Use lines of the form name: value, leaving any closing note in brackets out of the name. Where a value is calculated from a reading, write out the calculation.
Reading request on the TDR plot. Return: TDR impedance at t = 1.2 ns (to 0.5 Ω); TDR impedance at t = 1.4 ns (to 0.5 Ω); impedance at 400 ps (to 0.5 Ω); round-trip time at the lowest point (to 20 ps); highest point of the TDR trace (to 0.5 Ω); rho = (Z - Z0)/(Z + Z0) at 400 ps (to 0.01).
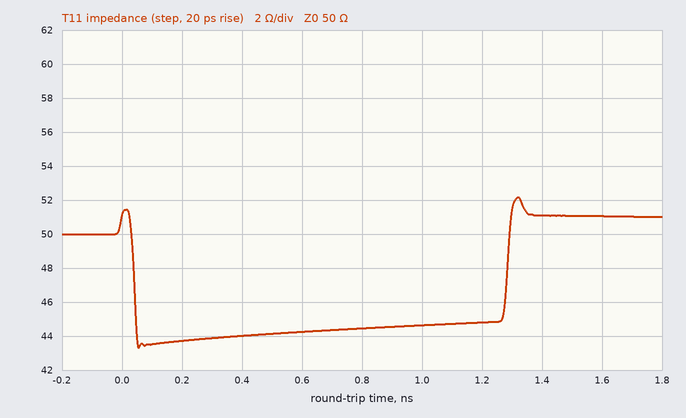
TDR impedance at t = 1.2 ns: 45.0 Ω
TDR impedance at t = 1.4 ns: 51.0 Ω
impedance at 400 ps: 44.0 Ω
round-trip time at the lowest point: 60 ps
highest point of the TDR trace: 52.0 Ω
rho = (Z - Z0)/(Z + Z0) at 400 ps: (44 − 50)/(44 + 50) ≈ -0.06
